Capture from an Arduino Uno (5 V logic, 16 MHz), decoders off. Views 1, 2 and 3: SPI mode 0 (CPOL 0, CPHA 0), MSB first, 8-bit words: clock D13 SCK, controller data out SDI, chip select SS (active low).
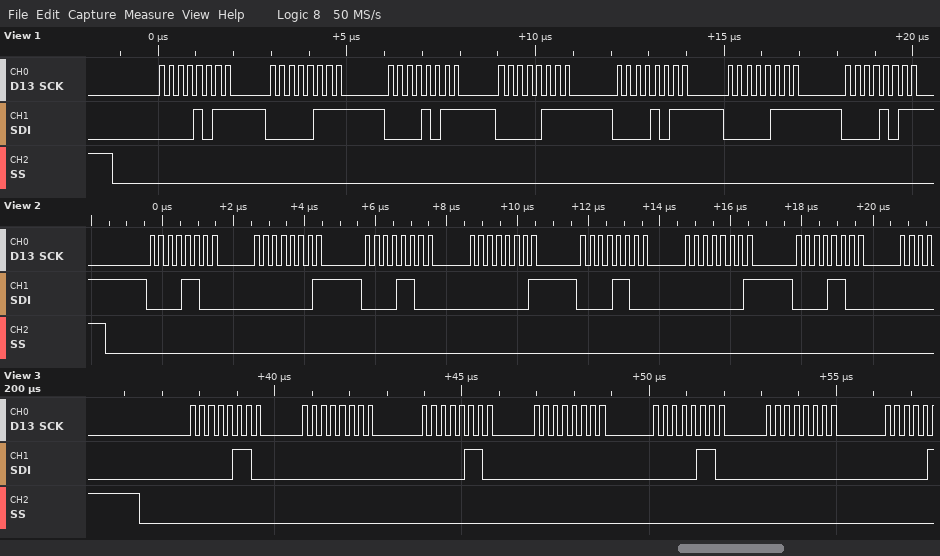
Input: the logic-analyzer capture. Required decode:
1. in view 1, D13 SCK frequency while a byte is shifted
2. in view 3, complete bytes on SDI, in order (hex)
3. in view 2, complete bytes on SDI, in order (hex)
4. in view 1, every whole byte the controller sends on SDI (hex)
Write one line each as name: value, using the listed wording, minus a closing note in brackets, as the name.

in view 1, D13 SCK frequency while a byte is shifted: 4 MHz
in view 3, complete bytes on SDI, in order: 0x06 0x00 0x06 0x00 0x06 0x00
in view 2, complete bytes on SDI, in order: 0C 01 0C 01 0C 01 0C
in view 1, every whole byte the controller sends on SDI: 0x0B 0x07 0x0B 0x07 0x0B 0x07 0x0B
